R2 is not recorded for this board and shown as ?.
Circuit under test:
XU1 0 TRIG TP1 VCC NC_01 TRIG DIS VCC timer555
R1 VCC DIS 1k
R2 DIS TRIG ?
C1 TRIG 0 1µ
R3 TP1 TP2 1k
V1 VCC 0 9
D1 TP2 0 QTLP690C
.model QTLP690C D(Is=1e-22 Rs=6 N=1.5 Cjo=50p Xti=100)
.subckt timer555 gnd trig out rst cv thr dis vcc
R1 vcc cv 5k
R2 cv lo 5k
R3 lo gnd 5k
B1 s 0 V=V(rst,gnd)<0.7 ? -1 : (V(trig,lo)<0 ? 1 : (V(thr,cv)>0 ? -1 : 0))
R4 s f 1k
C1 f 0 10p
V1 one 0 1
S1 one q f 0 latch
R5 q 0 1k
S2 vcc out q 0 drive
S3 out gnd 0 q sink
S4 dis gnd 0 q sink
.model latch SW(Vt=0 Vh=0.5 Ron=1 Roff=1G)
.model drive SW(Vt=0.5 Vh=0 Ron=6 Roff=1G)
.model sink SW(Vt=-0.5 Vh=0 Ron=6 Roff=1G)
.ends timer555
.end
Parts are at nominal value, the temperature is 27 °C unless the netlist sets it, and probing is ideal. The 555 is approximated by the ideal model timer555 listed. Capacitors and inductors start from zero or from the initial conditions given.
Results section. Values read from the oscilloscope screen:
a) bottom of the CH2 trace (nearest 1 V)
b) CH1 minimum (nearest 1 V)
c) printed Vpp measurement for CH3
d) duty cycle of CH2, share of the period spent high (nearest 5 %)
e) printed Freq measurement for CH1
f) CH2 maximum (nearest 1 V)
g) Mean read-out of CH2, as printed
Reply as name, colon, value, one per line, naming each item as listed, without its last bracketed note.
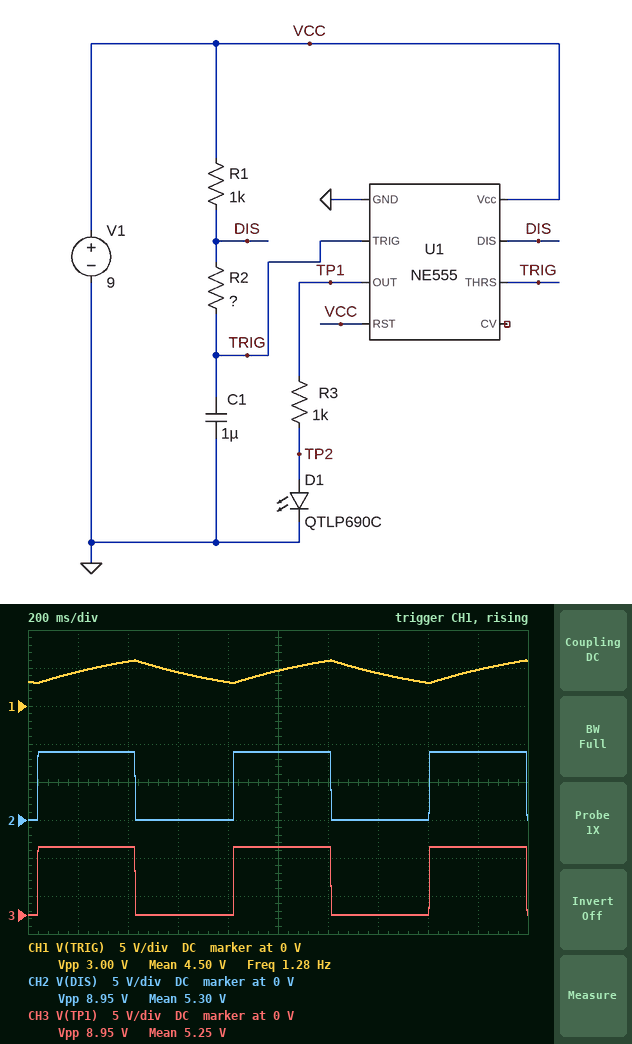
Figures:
bottom of the CH2 trace: 0 V
CH1 minimum: 3 V
printed Vpp measurement for CH3: 8.95 V
duty cycle of CH2, share of the period spent high: 50 %
printed Freq measurement for CH1: 1.28 Hz
CH2 maximum: 9 V
Mean read-out of CH2, as printed: 5.30 V
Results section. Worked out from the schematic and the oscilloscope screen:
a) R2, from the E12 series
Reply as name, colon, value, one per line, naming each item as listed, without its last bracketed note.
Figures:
R2, from the E12 series: 560 kΩ
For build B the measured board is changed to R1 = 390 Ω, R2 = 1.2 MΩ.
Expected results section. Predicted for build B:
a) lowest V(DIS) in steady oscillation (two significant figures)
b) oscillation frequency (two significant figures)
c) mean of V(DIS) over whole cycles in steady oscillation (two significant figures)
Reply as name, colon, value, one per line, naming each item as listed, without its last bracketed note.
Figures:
lowest V(DIS) in steady oscillation: 140 mV
oscillation frequency: 590 mHz
mean of V(DIS) over whole cycles in steady oscillation: 4.5 V
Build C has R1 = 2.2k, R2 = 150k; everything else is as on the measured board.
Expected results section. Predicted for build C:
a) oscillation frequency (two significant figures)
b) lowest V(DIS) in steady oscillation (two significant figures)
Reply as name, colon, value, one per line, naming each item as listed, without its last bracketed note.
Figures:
oscillation frequency: 4.8 Hz
lowest V(DIS) in steady oscillation: 25 mV
